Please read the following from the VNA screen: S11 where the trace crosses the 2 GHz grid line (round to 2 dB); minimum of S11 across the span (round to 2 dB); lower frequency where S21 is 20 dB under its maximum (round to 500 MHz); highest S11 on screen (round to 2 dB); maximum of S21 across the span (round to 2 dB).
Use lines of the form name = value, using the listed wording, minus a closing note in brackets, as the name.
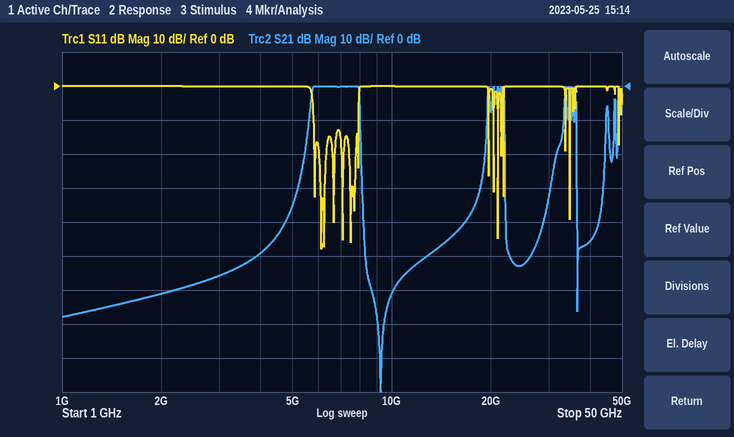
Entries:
S11 where the trace crosses the 2 GHz grid line = 0 dB
minimum of S11 across the span = -48 dB
lower frequency where S21 is 20 dB under its maximum = 5.5 GHz
highest S11 on screen = 0 dB
maximum of S21 across the span = 0 dB
